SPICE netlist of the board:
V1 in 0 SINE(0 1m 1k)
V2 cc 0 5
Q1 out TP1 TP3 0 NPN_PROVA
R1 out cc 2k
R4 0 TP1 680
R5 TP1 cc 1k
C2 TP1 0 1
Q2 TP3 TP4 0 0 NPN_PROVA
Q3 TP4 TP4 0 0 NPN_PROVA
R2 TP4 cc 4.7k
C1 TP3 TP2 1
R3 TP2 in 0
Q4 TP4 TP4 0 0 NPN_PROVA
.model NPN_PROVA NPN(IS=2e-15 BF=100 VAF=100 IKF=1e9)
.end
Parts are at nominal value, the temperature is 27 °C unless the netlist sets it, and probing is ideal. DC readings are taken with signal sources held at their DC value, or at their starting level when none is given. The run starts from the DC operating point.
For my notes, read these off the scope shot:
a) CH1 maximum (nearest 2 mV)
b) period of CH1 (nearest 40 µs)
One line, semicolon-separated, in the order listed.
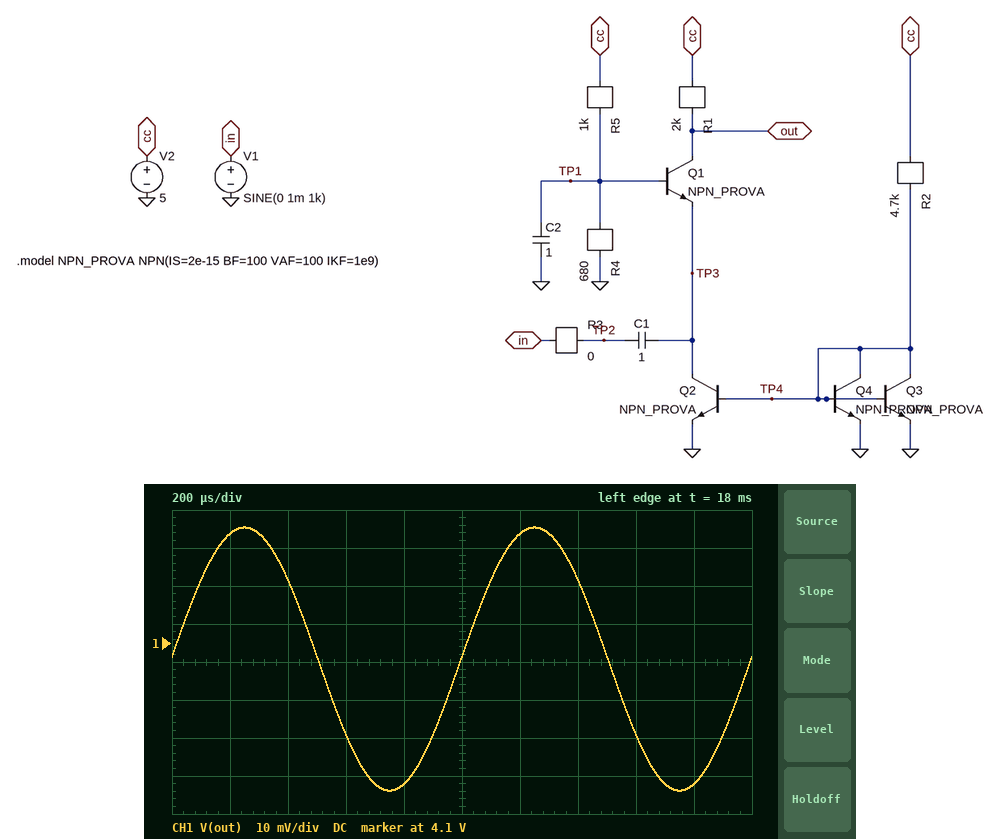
4.130 V; 1.00 ms
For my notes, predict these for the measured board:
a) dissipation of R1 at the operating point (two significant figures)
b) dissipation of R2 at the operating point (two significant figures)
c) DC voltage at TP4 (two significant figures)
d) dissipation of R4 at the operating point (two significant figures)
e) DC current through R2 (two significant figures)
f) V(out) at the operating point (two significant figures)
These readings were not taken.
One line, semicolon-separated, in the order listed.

410 µW; 4.0 mW; 680 mV; 6.0 mW; 920 µA; 4.1 V
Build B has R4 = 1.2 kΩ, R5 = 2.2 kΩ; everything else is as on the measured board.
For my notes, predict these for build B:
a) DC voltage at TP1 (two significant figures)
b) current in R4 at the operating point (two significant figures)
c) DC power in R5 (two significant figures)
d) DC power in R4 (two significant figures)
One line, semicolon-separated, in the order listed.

1.8 V; 1.5 mA; 4.8 mW; 2.6 mW
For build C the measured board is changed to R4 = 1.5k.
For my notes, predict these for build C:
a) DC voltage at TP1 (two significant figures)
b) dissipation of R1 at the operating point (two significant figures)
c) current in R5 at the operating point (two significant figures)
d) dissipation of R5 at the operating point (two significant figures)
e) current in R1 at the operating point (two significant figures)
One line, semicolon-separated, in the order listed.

3.0 V; 420 µW; 2.0 mA; 4.0 mW; 460 µA
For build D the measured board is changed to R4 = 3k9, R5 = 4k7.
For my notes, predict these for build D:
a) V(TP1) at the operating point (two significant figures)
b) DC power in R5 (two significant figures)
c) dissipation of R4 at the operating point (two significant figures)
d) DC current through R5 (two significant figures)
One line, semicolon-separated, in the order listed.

2.3 V; 1.6 mW; 1.3 mW; 580 µA
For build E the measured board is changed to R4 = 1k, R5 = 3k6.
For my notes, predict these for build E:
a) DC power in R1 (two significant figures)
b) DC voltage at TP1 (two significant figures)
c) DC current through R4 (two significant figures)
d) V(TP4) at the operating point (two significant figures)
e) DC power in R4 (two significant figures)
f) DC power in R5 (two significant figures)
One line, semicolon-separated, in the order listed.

400 µW; 1.1 V; 1.1 mA; 680 mV; 1.2 mW; 4.3 mW
